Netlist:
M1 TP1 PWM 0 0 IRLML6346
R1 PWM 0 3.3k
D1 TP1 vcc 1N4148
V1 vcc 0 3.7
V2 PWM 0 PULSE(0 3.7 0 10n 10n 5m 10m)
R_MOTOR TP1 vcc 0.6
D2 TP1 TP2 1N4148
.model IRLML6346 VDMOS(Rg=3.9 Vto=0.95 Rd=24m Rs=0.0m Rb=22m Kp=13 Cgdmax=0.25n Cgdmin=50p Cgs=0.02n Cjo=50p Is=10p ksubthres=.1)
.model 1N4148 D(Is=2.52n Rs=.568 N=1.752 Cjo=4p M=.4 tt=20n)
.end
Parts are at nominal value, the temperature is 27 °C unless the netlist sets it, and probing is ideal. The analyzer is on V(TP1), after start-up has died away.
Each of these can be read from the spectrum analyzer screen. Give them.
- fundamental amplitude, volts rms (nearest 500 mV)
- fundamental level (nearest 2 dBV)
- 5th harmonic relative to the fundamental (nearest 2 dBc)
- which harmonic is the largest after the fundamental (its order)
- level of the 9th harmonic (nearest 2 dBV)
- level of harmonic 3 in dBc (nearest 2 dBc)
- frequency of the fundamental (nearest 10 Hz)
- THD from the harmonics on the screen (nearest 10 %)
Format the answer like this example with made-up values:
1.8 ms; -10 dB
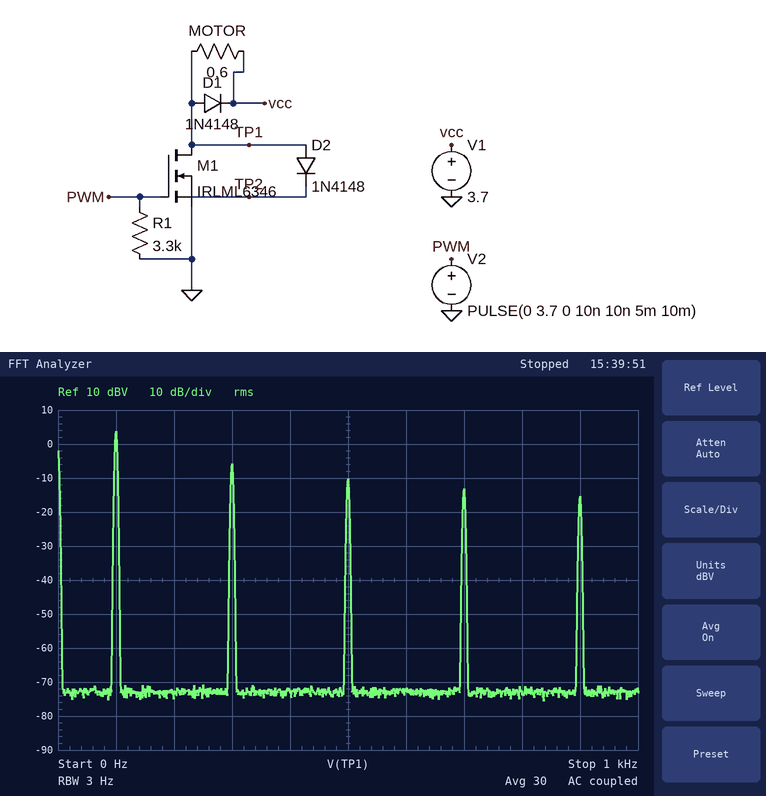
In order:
1.5 V; 4 dBV; -14 dBc; 3; -16 dBV; -10 dBc; 100 Hz; 40 %
